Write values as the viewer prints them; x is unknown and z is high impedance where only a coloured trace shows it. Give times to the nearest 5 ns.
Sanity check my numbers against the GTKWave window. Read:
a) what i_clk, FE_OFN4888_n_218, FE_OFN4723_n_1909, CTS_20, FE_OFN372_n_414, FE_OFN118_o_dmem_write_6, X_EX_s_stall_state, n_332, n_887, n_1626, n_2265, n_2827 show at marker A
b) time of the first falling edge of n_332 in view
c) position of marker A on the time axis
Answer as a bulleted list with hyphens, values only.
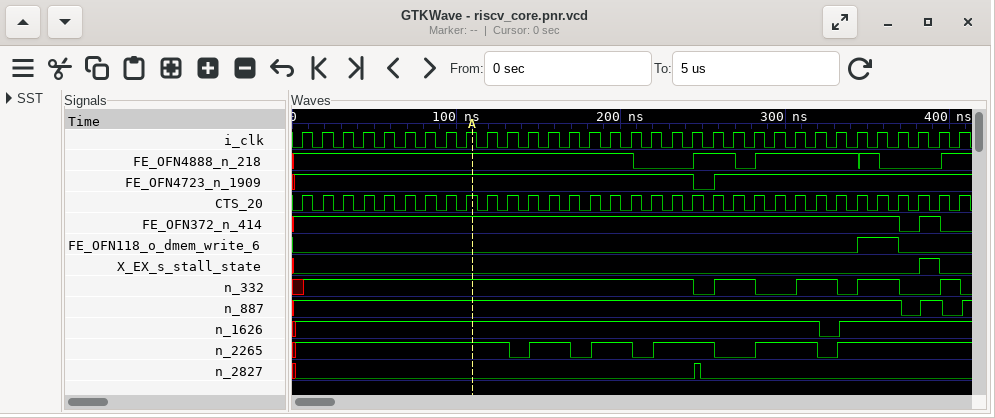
- i_clk=1, FE_OFN4888_n_218=1, FE_OFN4723_n_1909=1, CTS_20=1, FE_OFN372_n_414=1, FE_OFN118_o_dmem_write_6=0, X_EX_s_stall_state=0, n_332=1, n_887=1, n_1626=1, n_2265=1, n_2827=0
- 245 ns
- 110 ns
